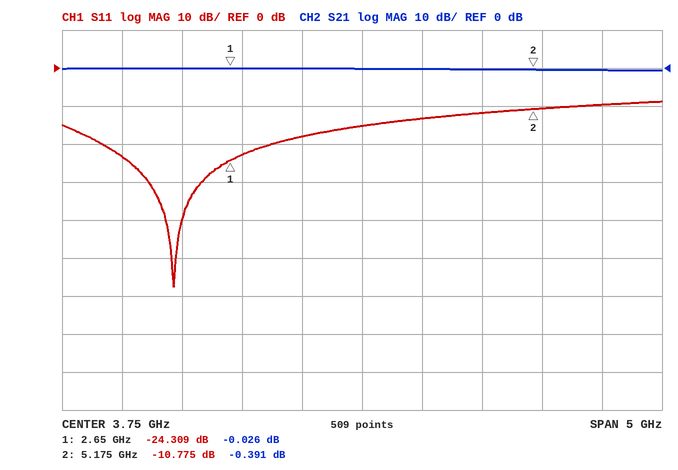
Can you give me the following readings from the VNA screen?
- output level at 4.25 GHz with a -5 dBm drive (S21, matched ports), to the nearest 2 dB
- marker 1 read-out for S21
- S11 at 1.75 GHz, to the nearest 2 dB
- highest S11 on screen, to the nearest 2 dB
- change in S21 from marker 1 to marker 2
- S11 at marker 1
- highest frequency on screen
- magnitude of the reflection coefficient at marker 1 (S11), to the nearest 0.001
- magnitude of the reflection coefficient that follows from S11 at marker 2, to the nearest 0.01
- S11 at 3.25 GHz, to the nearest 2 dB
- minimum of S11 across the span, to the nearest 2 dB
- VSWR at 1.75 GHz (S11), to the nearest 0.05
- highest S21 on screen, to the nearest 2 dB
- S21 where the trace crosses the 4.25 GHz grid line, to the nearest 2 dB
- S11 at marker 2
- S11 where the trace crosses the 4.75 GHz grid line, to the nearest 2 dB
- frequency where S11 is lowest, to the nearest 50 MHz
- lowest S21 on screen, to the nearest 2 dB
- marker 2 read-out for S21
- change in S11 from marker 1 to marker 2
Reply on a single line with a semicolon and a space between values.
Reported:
-6 dBm; -0.026 dB; -24 dB; -8 dB; -0.365 dB; -24.309 dB; 6.25 GHz; 0.061; 0.29; -18 dB; -58 dB; 1.15; 0 dB; 0 dB; -10.775 dB; -12 dB; 2.20 GHz; 0 dB; -0.391 dB; 13.534 dB
